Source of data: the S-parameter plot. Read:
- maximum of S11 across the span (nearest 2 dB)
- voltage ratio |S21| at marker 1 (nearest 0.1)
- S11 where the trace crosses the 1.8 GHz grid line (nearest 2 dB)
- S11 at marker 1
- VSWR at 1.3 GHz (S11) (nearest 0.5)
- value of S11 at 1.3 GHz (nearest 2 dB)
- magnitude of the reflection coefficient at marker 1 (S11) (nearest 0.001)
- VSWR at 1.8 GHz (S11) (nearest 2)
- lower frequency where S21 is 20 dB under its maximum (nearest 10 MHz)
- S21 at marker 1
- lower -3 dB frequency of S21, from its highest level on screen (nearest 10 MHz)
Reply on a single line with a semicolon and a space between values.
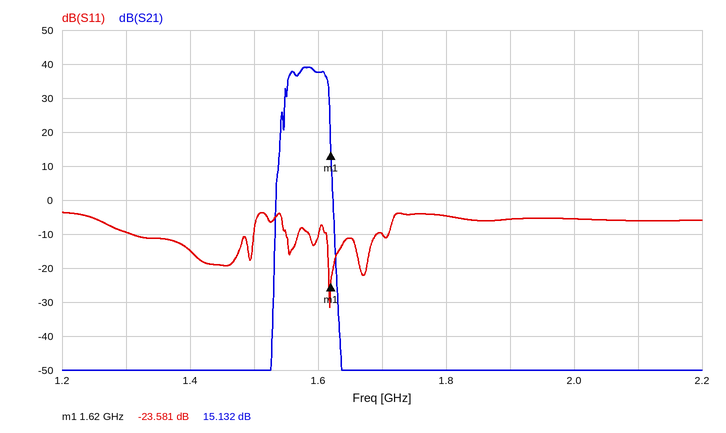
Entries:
-4 dB; 5.7; -4 dB; -23.581 dB; 2.0; -10 dB; 0.066; 4; 1.54 GHz; 15.132 dB; 1.55 GHz
